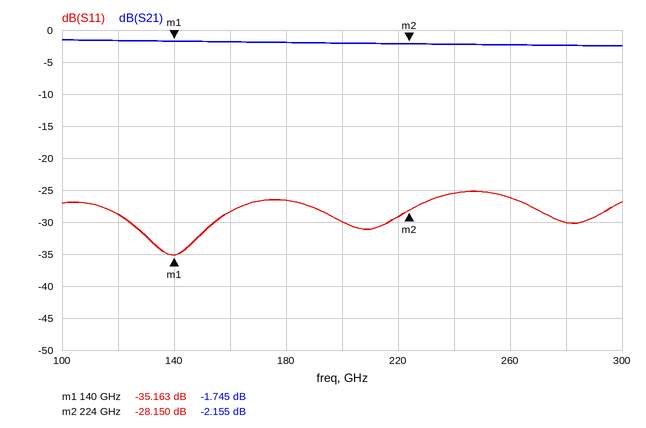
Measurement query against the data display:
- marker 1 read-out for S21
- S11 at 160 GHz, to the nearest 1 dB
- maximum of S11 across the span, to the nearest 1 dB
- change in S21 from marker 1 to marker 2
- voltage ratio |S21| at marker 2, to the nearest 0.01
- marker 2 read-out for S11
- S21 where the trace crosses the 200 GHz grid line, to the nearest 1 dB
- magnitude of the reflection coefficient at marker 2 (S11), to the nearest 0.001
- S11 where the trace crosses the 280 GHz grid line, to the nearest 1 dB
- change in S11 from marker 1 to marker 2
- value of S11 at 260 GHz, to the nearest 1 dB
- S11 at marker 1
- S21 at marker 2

-1.745 dB
-28 dB
-25 dB
-0.410 dB
0.78
-28.150 dB
-2 dB
0.039
-30 dB
7.013 dB
-26 dB
-35.163 dB
-2.155 dB
